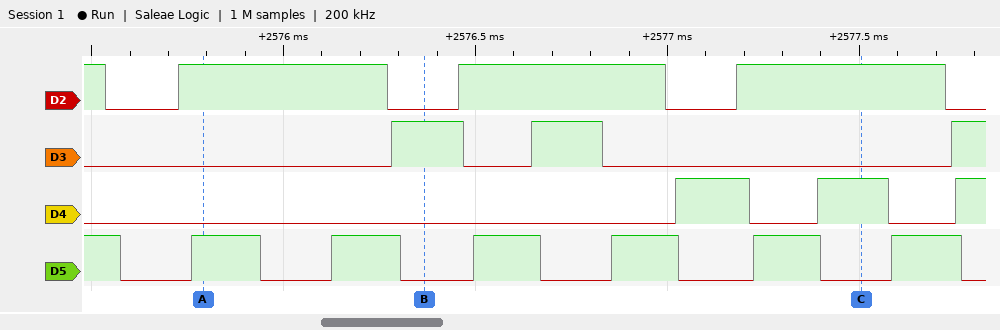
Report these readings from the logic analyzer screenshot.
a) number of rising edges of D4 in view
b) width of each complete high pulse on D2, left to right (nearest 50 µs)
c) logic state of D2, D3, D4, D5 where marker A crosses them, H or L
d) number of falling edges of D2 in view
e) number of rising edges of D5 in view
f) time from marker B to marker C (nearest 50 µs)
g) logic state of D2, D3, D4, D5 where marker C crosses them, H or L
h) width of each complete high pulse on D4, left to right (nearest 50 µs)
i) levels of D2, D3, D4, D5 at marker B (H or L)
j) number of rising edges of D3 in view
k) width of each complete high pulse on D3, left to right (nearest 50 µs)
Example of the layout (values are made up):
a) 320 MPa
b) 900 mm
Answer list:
a) 3
b) 550 µs, 550 µs, 550 µs
c) D2=H, D3=L, D4=L, D5=H
d) 4
e) 6
f) 1150 µs
g) D2=H, D3=L, D4=H, D5=L
h) 200 µs, 200 µs
i) D2=L, D3=H, D4=L, D5=L
j) 3
k) 200 µs, 200 µs
